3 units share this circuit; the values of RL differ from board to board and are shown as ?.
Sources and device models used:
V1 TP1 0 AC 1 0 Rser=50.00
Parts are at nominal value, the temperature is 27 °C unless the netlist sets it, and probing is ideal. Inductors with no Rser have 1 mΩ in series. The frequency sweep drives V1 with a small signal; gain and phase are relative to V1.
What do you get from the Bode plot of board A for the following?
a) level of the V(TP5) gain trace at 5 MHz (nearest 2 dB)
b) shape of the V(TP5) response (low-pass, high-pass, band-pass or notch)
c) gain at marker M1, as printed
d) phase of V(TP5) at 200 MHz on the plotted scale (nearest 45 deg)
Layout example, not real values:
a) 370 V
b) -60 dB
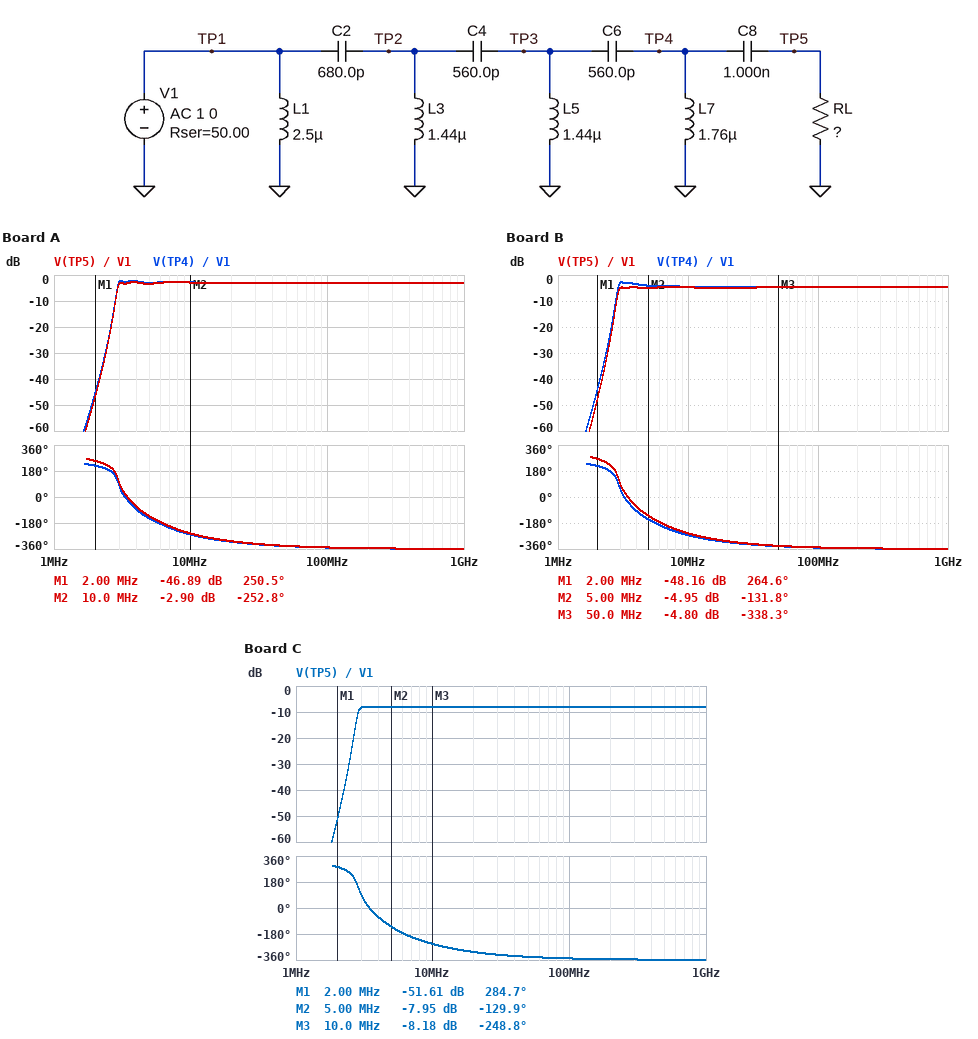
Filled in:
a) -4 dB
b) high-pass
c) -46.89 dB
d) -360 deg
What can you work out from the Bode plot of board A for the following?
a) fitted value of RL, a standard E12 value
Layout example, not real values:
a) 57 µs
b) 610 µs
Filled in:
a) 120 Ω
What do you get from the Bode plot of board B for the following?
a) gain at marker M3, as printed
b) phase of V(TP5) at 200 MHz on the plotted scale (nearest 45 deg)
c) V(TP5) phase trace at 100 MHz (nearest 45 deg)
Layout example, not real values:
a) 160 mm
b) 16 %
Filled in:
a) -4.80 dB
b) -360 deg
c) -360 deg
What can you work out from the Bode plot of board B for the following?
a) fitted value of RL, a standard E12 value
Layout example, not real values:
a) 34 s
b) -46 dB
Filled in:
a) 68 Ω
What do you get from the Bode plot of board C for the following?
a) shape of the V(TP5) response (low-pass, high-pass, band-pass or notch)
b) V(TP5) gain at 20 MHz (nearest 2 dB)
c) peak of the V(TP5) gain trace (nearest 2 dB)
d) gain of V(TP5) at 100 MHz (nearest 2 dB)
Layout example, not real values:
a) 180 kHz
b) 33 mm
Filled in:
a) high-pass
b) -8 dB
c) -8 dB
d) -8 dB
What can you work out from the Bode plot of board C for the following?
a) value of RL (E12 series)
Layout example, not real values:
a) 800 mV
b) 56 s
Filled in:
a) 33 Ω
